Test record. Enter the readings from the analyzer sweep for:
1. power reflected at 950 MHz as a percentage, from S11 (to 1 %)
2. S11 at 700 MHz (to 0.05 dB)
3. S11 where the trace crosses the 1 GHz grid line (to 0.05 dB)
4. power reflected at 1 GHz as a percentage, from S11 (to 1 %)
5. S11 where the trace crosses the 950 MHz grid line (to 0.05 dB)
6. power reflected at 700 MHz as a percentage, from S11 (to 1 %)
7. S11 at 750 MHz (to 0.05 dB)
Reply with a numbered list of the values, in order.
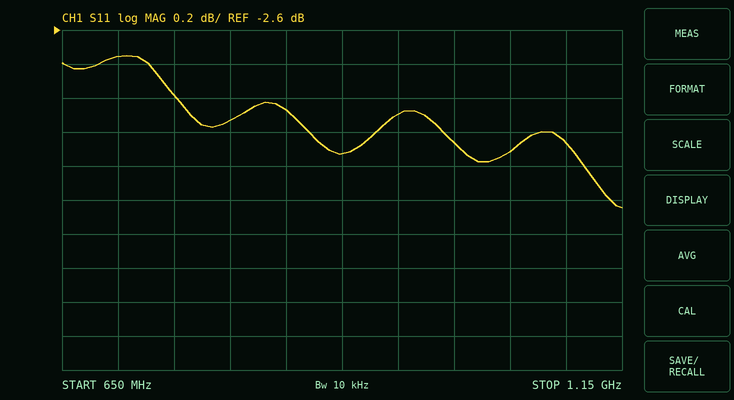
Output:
1. 49 %
2. -2.75 dB
3. -3.25 dB
4. 47 %
5. -3.10 dB
6. 53 %
7. -3.00 dB
